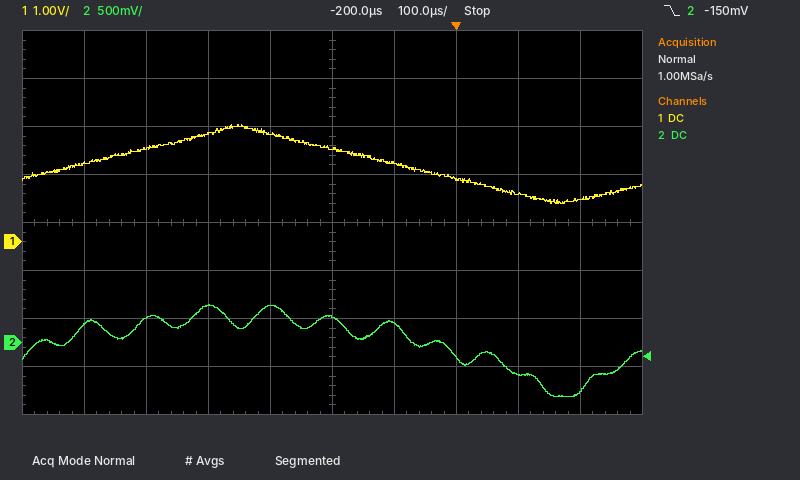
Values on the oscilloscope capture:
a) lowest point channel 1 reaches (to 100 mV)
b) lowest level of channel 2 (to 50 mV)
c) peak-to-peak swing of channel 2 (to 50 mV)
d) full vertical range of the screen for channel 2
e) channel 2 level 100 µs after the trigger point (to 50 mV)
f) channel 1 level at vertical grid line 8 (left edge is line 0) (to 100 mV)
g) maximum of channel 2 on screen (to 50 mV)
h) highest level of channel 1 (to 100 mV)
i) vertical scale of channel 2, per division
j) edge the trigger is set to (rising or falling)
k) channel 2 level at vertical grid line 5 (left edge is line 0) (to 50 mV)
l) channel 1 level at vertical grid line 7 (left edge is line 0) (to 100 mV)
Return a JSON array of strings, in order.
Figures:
["800 mV", "-550 mV", "950 mV", "4 V", "-350 mV", "1.0 V", "400 mV", "2.4 V", "500 mV", "falling", "250 mV", "1.3 V"]
